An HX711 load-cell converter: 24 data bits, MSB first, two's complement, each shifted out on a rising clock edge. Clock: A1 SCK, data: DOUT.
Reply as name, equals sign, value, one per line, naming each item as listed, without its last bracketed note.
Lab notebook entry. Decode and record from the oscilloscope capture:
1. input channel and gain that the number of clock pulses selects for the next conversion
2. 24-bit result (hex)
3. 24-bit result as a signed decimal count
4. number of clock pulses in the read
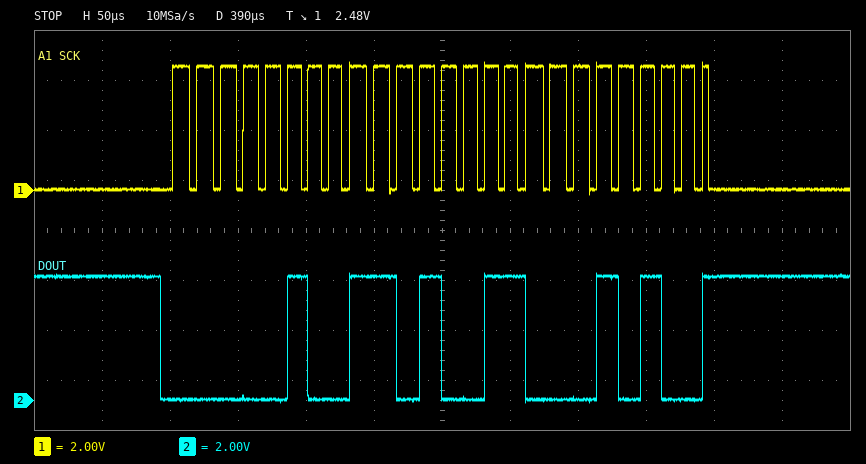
input channel and gain that the number of clock pulses selects for the next conversion = channel A, gain 128
24-bit result = 0x04D314
24-bit result as a signed decimal count = 316180
number of clock pulses in the read = 25
